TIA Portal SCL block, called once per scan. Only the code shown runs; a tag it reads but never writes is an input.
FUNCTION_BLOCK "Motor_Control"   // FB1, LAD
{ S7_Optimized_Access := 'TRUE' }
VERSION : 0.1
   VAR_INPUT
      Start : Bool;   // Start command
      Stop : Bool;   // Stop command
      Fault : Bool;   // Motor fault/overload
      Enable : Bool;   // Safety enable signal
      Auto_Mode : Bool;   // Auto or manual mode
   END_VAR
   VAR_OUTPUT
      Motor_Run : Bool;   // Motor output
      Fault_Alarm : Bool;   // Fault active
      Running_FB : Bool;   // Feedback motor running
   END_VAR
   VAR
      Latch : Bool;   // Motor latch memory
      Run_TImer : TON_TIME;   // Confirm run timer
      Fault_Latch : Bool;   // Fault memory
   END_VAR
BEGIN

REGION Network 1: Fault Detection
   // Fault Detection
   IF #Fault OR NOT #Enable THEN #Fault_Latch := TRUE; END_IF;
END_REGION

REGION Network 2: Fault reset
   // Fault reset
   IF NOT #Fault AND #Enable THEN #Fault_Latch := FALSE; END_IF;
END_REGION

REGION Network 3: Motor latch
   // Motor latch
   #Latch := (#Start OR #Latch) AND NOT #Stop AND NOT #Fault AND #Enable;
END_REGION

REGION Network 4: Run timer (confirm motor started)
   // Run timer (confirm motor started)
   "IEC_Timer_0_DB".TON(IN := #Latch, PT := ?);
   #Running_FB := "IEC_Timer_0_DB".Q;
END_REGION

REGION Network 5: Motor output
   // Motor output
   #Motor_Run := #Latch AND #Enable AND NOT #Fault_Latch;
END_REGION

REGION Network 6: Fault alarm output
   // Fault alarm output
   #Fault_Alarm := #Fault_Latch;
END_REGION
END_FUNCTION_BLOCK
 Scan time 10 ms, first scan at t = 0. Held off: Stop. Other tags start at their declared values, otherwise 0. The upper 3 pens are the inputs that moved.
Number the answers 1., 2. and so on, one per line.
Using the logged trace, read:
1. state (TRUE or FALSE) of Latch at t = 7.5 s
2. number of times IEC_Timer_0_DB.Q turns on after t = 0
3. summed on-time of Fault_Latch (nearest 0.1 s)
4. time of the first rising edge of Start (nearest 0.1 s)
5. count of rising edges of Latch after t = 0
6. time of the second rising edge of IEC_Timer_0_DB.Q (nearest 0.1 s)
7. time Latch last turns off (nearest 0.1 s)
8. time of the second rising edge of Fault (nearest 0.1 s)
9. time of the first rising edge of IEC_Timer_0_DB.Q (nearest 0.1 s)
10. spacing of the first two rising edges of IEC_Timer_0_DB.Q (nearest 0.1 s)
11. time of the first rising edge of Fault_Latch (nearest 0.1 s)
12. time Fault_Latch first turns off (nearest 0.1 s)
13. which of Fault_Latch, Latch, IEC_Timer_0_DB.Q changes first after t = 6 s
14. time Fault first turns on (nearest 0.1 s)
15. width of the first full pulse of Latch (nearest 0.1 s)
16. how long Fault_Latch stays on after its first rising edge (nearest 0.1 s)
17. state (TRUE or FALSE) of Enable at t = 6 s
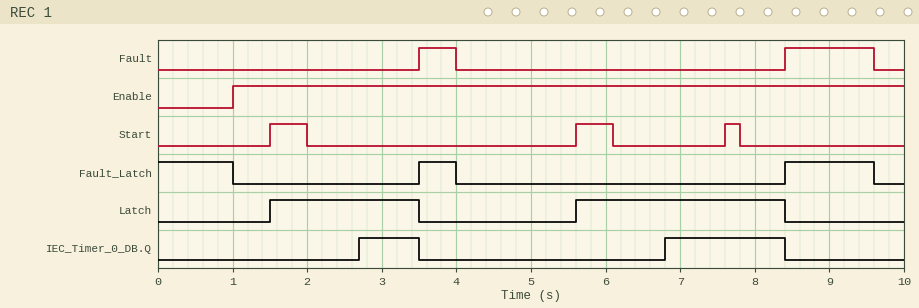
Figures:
1. TRUE
2. 2
3. 2.7 s
4. 1.5 s
5. 2
6. 6.8 s
7. 8.4 s
8. 8.4 s
9. 2.7 s
10. 4.1 s
11. 3.5 s
12. 1.0 s
13. IEC_Timer_0_DB.Q
14. 3.5 s
15. 2.0 s
16. 0.5 s
17. TRUE
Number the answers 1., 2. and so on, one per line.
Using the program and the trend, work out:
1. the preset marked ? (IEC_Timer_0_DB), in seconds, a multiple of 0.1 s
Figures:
1. 1.2 s
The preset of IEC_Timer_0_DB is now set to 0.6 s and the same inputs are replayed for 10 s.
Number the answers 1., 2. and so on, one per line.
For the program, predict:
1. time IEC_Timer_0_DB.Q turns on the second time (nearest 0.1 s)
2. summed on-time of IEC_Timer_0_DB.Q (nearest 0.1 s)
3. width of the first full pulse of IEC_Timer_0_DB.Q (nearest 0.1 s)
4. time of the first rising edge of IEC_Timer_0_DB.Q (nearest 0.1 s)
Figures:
1. 6.2 s
2. 3.6 s
3. 1.4 s
4. 2.1 s
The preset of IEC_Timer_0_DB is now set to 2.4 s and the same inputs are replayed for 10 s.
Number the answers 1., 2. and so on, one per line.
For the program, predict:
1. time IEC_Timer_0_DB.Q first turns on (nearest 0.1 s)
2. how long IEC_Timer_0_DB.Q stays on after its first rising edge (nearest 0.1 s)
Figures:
1. 8.0 s
2. 0.4 s
